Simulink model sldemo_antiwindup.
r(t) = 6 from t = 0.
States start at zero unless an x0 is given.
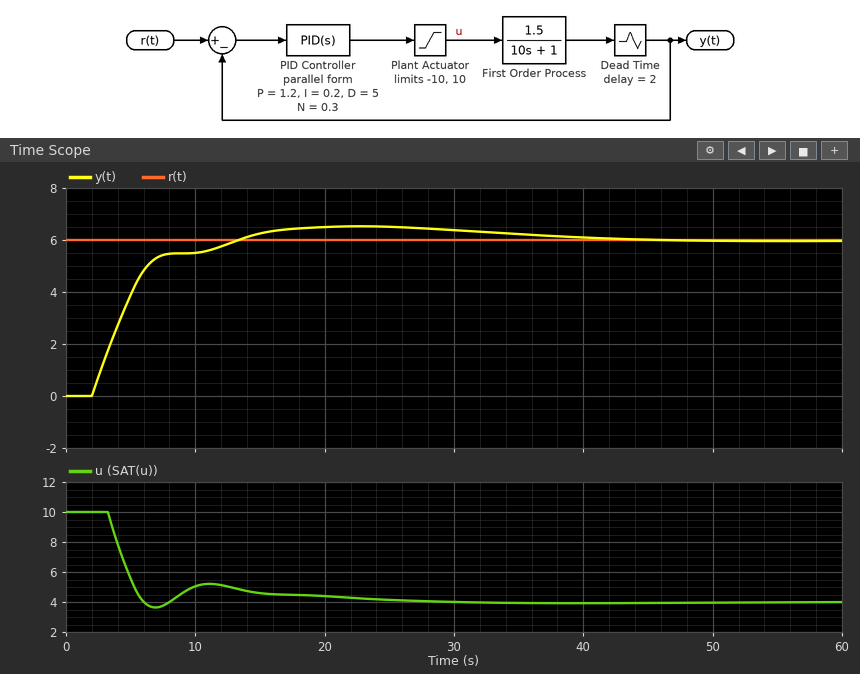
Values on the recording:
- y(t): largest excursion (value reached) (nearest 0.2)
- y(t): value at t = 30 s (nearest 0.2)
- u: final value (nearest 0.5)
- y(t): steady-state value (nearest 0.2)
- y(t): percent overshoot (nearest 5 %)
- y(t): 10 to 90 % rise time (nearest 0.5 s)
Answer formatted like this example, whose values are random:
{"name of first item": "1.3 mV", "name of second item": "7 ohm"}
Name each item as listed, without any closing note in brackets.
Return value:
{"y(t): largest excursion (value reached)": "6.6", "y(t): value at t = 30 s": "6.4", "u: final value": "4.0", "y(t): steady-state value": "6.0", "y(t): percent overshoot": "10 %", "y(t): 10 to 90 % rise time": "5.0 s"}
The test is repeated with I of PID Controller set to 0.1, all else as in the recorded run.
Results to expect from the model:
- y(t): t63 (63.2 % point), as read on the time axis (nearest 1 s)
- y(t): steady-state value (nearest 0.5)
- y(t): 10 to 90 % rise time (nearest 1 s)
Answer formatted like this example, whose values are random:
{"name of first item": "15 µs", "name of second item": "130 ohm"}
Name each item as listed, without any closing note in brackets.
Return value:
{"y(t): t63 (63.2 % point), as read on the time axis": "5 s", "y(t): steady-state value": "6.0", "y(t): 10 to 90 % rise time": "15 s"}
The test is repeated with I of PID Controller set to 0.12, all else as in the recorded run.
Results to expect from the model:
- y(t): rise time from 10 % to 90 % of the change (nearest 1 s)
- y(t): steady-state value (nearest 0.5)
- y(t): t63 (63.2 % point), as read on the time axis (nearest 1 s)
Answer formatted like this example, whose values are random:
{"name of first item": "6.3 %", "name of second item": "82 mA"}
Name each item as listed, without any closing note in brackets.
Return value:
{"y(t): rise time from 10 % to 90 % of the change": "12 s", "y(t): steady-state value": "6.0", "y(t): t63 (63.2 % point), as read on the time axis": "5 s"}
